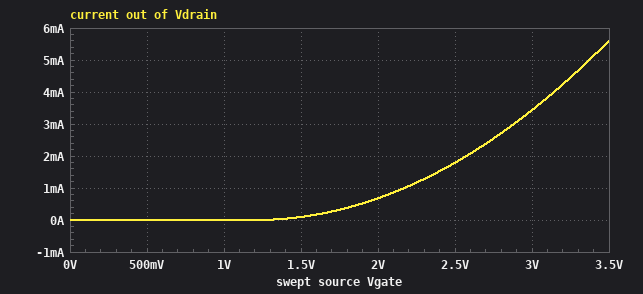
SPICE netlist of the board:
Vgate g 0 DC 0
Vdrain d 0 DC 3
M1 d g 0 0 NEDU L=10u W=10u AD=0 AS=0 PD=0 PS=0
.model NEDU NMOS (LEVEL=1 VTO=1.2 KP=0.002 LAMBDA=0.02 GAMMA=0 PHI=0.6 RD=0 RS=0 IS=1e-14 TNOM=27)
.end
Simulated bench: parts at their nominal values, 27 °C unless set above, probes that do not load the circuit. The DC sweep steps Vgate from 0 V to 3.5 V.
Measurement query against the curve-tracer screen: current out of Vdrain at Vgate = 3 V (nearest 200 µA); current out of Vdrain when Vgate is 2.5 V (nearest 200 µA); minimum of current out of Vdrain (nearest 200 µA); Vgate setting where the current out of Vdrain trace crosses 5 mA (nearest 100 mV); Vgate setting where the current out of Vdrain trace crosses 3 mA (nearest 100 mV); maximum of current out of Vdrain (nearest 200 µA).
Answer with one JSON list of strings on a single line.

["3.4 mA", "1.8 mA", "0 A", "3.4 V", "2.9 V", "5.6 mA"]
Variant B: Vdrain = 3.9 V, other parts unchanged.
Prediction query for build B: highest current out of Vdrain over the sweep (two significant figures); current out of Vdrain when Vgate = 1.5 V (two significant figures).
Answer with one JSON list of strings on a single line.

["5.7 mA", "97 µA"]
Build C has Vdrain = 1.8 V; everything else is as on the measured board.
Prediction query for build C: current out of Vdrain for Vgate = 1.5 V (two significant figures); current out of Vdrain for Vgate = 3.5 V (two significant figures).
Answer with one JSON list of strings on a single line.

["93 µA", "5.2 mA"]
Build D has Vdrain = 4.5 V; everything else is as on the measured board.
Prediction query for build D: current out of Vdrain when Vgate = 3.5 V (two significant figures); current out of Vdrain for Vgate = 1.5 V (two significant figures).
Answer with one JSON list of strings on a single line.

["5.8 mA", "98 µA"]
